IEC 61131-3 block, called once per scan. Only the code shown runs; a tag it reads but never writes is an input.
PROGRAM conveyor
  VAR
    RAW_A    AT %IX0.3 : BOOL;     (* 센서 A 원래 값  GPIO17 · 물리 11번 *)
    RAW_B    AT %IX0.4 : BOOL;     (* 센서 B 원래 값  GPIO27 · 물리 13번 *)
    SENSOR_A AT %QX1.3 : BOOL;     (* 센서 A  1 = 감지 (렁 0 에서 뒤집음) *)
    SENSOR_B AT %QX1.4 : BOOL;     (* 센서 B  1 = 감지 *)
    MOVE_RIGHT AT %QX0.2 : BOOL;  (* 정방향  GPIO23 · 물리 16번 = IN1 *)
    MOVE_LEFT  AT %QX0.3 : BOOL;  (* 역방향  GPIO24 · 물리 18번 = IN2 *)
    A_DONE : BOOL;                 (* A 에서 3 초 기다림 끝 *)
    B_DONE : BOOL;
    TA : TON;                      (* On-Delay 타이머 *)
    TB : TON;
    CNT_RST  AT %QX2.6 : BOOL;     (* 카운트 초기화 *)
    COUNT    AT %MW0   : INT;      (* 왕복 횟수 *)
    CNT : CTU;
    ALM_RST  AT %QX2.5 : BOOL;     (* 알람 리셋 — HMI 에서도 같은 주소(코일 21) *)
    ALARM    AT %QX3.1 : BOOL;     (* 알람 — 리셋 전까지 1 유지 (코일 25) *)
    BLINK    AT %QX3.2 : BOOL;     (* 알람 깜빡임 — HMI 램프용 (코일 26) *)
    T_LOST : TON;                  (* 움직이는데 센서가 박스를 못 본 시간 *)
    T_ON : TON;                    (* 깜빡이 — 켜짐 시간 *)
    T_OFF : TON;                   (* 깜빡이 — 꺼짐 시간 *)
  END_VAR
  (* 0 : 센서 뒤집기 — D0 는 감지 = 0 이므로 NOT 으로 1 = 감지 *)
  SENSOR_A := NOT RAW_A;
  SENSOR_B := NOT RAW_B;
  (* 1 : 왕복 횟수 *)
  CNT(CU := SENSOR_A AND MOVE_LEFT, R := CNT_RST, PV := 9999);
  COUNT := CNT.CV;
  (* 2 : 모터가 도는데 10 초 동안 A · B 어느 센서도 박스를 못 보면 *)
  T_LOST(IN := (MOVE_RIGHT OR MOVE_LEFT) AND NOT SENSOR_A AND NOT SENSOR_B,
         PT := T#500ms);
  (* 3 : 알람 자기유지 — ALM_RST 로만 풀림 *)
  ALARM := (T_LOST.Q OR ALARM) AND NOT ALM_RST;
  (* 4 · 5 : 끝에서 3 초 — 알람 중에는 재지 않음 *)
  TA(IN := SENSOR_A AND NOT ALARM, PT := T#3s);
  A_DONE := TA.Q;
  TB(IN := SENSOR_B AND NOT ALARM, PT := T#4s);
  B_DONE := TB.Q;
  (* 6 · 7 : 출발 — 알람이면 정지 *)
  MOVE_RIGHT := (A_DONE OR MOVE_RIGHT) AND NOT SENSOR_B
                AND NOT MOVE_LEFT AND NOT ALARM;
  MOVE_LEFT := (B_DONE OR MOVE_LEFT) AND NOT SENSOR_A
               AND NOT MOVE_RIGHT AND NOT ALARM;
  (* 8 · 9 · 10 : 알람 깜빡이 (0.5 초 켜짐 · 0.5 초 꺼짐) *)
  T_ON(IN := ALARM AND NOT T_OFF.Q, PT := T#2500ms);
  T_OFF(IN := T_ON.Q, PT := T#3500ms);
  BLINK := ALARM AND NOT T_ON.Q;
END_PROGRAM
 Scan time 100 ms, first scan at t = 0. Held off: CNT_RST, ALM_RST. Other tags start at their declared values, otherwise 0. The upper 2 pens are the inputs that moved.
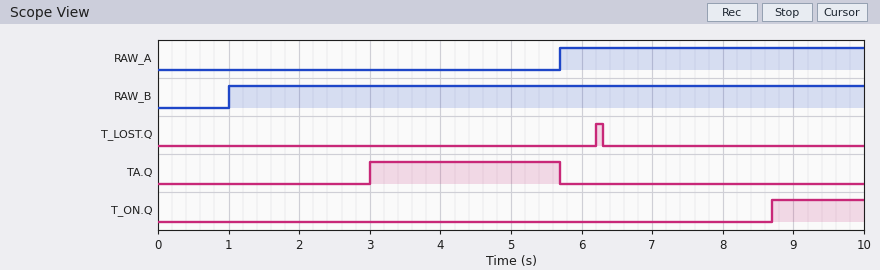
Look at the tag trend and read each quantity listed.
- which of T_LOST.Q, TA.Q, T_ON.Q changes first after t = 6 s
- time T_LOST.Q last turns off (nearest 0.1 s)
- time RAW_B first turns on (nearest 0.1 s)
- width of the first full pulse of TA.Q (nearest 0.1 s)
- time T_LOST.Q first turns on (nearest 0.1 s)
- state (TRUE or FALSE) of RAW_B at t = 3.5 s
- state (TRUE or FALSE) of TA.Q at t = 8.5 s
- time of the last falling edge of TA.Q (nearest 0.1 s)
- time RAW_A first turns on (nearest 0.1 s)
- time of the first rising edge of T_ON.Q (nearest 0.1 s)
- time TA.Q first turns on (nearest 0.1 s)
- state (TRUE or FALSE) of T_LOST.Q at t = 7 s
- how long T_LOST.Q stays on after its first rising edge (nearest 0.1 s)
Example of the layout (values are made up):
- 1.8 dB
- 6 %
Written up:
- T_LOST.Q
- 6.3 s
- 1.0 s
- 2.7 s
- 6.2 s
- TRUE
- FALSE
- 5.7 s
- 5.7 s
- 8.7 s
- 3.0 s
- FALSE
- 0.1 s
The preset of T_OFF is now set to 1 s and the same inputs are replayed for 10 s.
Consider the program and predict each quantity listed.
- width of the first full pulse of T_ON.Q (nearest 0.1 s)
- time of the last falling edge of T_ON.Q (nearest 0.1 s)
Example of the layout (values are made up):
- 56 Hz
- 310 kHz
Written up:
- 1.1 s
- 9.8 s
